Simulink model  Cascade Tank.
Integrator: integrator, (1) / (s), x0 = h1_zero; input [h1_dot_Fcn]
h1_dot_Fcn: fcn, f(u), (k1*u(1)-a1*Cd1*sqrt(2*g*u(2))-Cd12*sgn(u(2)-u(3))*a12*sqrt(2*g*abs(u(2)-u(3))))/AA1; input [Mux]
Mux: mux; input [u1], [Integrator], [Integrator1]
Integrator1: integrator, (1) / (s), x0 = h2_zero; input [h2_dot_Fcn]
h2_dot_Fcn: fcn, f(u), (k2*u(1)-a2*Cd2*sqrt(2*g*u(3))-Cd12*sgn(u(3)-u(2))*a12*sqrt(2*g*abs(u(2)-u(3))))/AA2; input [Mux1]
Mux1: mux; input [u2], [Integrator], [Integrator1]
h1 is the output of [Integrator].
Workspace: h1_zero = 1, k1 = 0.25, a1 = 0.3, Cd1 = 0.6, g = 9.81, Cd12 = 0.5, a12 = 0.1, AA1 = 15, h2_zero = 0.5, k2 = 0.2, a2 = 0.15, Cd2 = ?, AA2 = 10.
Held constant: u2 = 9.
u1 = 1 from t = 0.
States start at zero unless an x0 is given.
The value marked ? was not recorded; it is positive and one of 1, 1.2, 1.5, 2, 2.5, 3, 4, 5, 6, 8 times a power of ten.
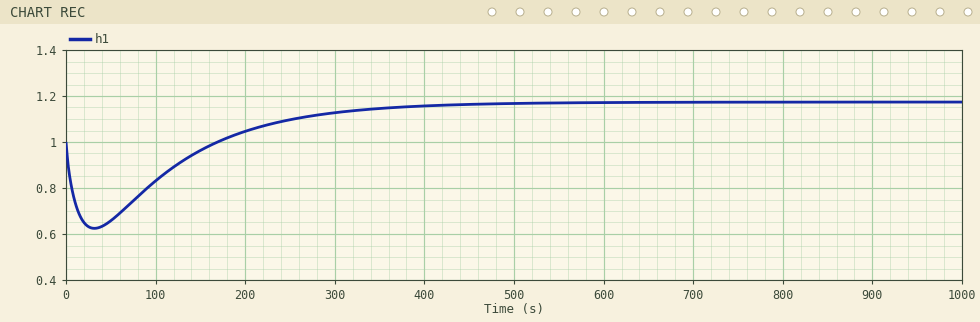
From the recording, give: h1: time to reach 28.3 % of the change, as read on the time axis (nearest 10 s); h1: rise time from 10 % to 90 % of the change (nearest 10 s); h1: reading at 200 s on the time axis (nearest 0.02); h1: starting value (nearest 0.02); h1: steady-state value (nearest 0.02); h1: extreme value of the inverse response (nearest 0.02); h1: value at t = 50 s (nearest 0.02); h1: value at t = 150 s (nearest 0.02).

200 s
220 s
1.04
1.00
1.18
0.62
0.66
0.96
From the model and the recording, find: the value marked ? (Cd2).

0.6
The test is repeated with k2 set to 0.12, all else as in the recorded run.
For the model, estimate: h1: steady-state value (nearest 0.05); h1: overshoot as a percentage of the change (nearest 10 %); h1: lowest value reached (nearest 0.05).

0.60
30 %
0.50
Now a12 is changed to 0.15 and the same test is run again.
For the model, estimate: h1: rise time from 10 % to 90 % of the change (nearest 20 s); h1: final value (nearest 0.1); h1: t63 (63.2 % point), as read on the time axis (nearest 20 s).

180 s
1.6
160 s
